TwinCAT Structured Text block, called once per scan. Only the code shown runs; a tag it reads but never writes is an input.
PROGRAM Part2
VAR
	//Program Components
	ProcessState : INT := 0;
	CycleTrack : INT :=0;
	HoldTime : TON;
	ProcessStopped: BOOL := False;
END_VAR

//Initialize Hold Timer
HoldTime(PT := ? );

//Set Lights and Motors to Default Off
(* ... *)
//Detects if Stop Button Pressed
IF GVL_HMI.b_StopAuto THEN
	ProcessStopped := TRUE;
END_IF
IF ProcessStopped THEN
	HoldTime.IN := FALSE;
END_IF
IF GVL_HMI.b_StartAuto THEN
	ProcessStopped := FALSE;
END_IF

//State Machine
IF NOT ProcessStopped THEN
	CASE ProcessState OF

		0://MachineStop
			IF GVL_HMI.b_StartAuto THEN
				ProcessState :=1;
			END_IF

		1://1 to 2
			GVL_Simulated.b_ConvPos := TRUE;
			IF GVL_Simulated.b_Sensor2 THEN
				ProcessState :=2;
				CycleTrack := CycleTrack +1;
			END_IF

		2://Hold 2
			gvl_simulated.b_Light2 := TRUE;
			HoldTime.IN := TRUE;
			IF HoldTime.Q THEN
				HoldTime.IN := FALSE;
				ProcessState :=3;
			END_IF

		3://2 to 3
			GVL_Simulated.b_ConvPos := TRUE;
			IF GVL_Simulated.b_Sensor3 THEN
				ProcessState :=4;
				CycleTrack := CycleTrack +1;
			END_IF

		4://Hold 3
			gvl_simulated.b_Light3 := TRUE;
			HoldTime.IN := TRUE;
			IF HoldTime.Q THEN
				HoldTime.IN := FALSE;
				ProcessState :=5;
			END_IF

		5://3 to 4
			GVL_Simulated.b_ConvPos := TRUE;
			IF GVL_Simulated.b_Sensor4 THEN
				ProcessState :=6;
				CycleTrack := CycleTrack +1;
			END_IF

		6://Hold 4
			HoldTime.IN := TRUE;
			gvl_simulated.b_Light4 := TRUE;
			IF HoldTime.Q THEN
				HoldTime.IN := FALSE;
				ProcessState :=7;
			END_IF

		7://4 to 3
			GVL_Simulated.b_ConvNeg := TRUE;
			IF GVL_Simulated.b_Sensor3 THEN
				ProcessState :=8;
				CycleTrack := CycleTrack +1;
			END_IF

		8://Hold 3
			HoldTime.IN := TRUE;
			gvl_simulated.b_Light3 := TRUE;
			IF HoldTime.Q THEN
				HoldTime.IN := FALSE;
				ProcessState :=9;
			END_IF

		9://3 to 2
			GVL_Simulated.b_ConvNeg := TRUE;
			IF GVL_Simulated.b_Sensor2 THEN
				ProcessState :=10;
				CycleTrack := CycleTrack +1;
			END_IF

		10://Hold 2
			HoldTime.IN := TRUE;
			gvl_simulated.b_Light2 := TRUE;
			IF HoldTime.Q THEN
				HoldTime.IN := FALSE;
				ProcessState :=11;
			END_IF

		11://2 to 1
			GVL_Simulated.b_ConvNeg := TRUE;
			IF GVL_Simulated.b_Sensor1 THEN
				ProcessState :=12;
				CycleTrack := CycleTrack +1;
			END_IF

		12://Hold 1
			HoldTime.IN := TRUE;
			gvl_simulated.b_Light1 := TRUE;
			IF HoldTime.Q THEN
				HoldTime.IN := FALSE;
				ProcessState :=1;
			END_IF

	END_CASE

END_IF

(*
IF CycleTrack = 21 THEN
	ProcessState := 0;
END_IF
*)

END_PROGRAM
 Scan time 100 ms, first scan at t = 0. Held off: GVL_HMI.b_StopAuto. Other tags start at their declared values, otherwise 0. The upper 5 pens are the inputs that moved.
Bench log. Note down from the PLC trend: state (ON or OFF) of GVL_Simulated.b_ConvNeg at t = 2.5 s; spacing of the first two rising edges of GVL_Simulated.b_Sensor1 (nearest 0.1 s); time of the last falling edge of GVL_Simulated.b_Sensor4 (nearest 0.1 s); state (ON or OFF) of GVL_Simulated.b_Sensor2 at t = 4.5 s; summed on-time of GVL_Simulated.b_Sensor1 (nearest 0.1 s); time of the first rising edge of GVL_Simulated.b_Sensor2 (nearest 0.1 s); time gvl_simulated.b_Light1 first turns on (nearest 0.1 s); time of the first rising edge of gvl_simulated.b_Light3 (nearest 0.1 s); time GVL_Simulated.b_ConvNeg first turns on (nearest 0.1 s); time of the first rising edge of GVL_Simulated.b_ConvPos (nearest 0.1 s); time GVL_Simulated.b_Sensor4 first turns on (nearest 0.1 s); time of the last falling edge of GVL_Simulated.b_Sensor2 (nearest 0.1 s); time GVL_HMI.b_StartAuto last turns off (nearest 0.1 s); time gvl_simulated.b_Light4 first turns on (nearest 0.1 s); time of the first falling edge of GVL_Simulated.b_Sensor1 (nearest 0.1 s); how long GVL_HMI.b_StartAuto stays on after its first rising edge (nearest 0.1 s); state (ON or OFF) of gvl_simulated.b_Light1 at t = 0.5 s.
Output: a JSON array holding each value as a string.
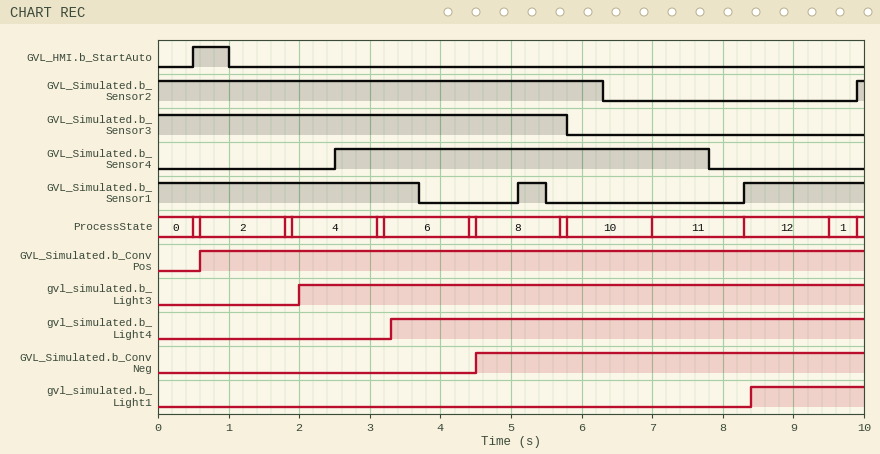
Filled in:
["OFF", "3.2 s", "7.8 s", "ON", "5.8 s", "9.9 s", "8.4 s", "2.0 s", "4.5 s", "0.6 s", "2.5 s", "6.3 s", "1.0 s", "3.3 s", "3.7 s", "0.5 s", "OFF"]
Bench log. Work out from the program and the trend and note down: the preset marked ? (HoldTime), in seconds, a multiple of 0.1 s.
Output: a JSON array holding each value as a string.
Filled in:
["1.0 s"]
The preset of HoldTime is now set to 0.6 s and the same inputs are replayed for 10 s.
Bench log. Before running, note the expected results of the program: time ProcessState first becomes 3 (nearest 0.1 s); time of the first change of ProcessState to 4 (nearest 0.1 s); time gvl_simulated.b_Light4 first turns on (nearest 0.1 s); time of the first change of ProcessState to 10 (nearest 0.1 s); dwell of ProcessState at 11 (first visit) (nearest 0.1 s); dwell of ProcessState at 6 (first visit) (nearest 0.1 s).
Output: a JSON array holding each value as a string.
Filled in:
["1.4 s", "1.5 s", "2.6 s", "4.3 s", "0.1 s", "0.8 s"]
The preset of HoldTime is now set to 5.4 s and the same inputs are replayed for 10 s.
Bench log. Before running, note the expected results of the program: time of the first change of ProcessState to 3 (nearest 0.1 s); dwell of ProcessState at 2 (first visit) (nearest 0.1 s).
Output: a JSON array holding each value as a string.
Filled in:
["6.2 s", "5.6 s"]
